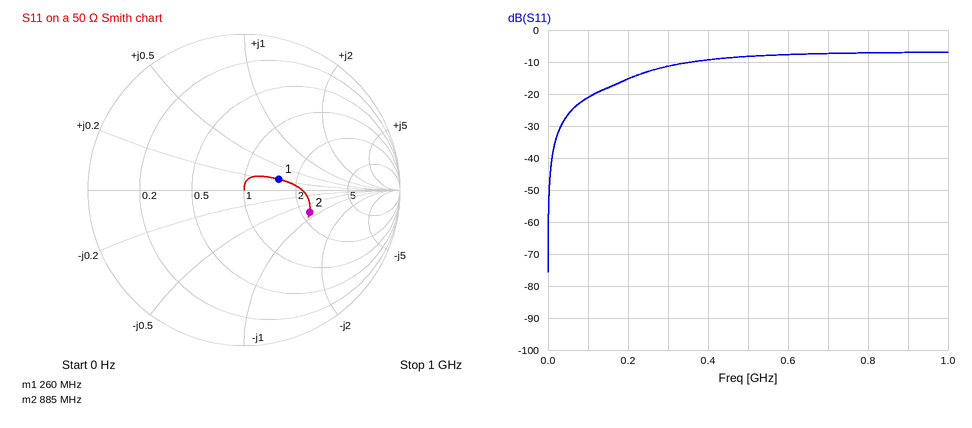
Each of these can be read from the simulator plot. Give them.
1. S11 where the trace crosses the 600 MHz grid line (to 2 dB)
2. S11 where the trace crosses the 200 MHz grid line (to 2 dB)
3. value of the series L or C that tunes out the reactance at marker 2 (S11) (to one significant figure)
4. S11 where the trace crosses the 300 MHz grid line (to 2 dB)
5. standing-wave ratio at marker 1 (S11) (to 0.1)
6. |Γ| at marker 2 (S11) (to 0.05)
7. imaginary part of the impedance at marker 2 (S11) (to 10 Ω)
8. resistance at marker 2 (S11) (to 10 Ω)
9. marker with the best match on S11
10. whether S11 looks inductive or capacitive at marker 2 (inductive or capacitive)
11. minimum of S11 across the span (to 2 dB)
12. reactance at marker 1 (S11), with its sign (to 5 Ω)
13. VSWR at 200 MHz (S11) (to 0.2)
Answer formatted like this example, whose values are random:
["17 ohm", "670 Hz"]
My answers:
["-8 dB", "-16 dB", "7 nH", "-12 dB", "1.6", "0.45", "-40 Ω", "110 Ω", "marker 1", "capacitive", "-76 dB", "+10 Ω", "1.4"]
